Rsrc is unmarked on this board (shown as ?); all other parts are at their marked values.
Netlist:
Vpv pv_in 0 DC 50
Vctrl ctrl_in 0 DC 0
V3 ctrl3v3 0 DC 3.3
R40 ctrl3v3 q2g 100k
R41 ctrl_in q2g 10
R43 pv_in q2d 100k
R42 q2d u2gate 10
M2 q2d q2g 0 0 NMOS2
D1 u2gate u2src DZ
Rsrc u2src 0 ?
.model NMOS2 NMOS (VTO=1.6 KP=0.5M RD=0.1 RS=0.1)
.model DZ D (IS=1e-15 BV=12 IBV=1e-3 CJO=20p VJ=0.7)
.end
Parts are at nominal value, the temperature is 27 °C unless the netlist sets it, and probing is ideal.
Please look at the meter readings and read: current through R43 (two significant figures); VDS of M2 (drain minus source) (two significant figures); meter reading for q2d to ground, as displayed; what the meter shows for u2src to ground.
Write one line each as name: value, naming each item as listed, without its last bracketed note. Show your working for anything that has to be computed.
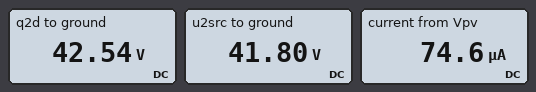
current through R43: (50 V - 42.54 V) / 100 kΩ = 75 µA
VDS of M2 (drain minus source): 42.54 V = 43 V
meter reading for q2d to ground, as displayed: 42.54 V
what the meter shows for u2src to ground: 41.80 V
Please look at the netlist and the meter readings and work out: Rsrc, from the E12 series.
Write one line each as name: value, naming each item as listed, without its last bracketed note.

Rsrc, from the E12 series: 560 kΩ
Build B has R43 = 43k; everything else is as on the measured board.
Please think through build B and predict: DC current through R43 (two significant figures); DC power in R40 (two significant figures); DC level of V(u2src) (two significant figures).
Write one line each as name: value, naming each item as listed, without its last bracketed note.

DC current through R43: 82 µA
DC power in R40: 110 µW
DC level of V(u2src): 46 V
